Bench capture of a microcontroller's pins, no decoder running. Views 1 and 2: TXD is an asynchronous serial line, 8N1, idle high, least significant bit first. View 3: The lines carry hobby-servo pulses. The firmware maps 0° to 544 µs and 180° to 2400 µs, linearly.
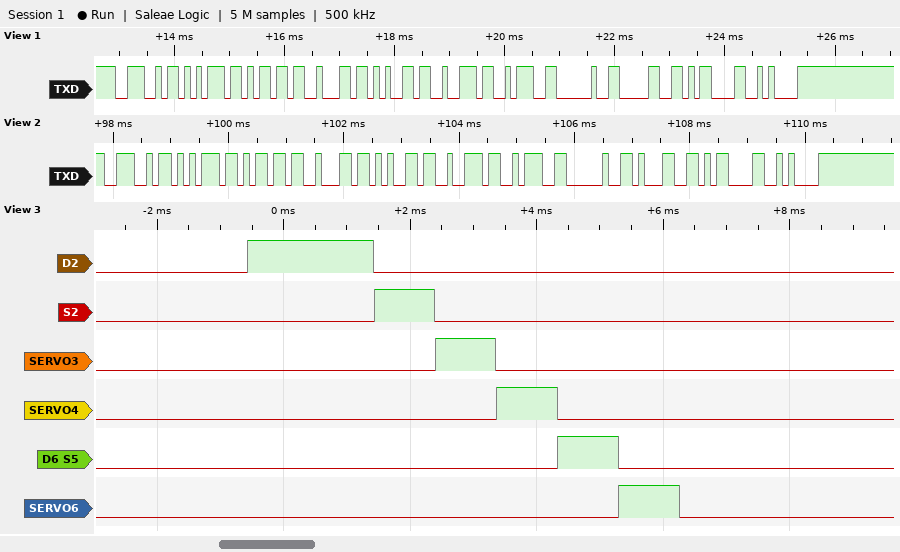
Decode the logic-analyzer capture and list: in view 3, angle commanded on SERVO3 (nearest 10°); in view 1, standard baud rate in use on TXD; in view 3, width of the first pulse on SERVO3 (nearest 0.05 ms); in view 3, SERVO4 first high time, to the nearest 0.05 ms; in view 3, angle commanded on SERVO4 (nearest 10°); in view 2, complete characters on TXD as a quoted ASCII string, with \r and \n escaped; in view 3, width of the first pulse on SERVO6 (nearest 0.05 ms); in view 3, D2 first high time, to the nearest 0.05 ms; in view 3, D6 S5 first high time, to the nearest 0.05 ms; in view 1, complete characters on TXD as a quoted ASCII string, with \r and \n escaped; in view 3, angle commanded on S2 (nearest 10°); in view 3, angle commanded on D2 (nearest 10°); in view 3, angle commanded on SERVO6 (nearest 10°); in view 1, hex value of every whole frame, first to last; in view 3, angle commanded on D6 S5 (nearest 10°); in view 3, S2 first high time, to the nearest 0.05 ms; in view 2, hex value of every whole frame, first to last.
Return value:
40°
9600 baud
0.95 ms
0.95 ms
40°
"Number: 1\r\n"
0.95 ms
2.00 ms
0.95 ms
"Number: 0\r\n"
40°
140°
40°
4E 75 6D 62 65 72 3A 20 30 0D 0A
40°
0.95 ms
4E 75 6D 62 65 72 3A 20 31 0D 0A
